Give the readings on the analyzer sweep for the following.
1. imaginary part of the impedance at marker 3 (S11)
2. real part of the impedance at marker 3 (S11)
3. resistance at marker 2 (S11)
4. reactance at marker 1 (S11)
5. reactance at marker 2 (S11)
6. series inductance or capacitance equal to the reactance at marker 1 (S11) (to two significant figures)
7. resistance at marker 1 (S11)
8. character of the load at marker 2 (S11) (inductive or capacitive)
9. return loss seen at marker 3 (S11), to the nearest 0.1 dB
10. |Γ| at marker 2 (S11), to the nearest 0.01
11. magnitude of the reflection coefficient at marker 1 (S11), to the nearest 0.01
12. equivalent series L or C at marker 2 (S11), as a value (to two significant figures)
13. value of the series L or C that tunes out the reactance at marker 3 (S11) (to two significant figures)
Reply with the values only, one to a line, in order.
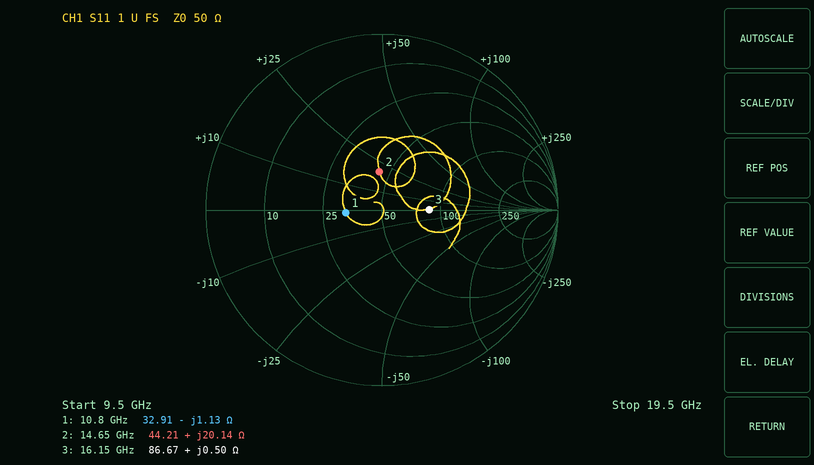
+0.50 Ω
86.67 Ω
44.21 Ω
-1.13 Ω
+20.14 Ω
13 pF
32.91 Ω
inductive
11.4 dB
0.22
0.21
220 pH
20 pF
